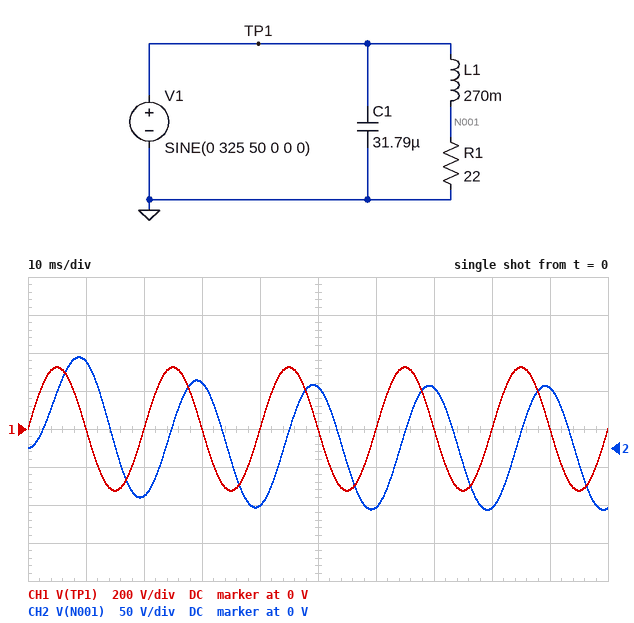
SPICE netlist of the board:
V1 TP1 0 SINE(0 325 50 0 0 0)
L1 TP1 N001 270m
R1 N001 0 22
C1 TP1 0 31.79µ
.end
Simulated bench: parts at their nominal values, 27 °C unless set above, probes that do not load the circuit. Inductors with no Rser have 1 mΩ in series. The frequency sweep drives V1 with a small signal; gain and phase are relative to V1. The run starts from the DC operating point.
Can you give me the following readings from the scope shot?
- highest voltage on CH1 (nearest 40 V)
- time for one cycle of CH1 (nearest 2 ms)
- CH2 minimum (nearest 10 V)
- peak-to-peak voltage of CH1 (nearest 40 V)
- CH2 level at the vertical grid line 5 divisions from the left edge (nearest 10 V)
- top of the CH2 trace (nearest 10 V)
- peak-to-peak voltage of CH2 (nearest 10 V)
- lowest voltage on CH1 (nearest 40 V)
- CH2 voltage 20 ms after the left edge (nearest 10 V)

320 V
20 ms
-80 V
640 V
80 V
120 V
200 V
-320 V
-60 V
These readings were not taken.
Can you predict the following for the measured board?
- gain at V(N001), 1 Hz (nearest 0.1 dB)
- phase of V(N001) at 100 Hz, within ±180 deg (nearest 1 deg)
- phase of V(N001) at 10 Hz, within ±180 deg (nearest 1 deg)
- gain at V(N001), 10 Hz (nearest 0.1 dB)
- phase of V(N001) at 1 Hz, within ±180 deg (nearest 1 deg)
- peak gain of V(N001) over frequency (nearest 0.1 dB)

0 dB
-83 deg
-38 deg
-2.0 dB
-4 deg
0 dB
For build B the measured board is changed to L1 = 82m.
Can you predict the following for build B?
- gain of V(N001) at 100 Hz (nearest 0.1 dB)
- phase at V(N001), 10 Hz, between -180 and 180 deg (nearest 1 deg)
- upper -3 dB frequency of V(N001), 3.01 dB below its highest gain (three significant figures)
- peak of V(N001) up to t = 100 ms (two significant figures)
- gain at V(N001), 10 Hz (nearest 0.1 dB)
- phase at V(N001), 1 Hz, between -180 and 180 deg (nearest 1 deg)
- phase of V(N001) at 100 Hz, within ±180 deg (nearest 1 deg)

-8.1 dB
-13 deg
42.7 Hz
230 V
-0.2 dB
-1 deg
-67 deg
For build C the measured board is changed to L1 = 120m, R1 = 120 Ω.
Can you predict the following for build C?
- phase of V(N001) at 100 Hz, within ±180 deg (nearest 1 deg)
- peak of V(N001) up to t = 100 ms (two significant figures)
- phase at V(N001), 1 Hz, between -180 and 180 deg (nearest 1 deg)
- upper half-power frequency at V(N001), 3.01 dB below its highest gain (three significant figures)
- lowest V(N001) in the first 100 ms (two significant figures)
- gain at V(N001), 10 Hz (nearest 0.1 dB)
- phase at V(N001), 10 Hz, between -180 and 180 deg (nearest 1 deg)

-32 deg
310 V
0 deg
159 Hz
-310 V
0 dB
-4 deg
